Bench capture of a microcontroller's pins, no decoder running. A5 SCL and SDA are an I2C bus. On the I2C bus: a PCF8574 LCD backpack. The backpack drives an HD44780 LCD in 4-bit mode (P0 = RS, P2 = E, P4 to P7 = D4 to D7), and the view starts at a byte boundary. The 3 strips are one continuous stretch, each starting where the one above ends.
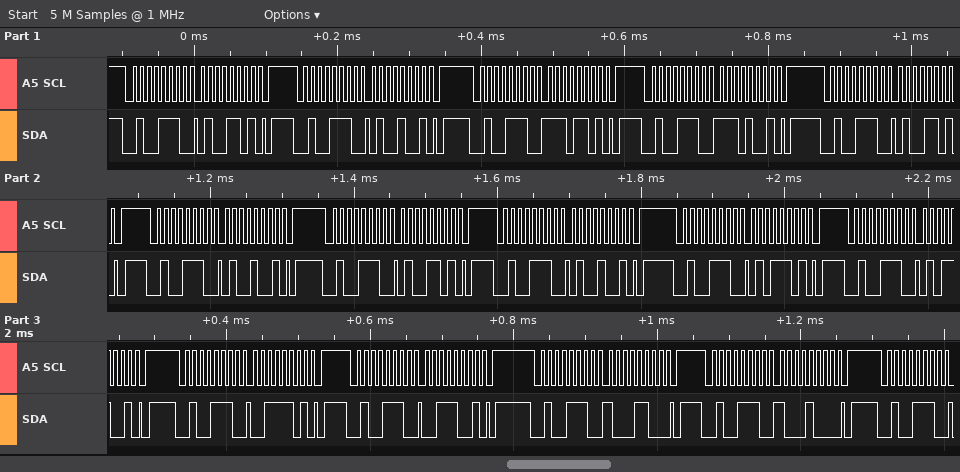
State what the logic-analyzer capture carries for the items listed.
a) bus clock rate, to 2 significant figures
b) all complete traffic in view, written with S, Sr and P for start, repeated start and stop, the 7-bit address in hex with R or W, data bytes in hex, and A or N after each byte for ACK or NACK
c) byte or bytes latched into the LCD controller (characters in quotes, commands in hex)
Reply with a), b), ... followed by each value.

a) 100 kHz
b) S 27W A 4D A P S 27W A 49 A P S 27W A ED A P S 27W A E9 A P S 27W A 4D A P S 27W A 49 A P S 27W A 4D A P S 27W A 49 A P S 27W A 5D A P S 27W A 59 A P S 27W A 3D A P S 27W A 39 A P S 27W A 8C A P S 27W A 88 A P S 27W A
c) 'N' 'D' 'S'
